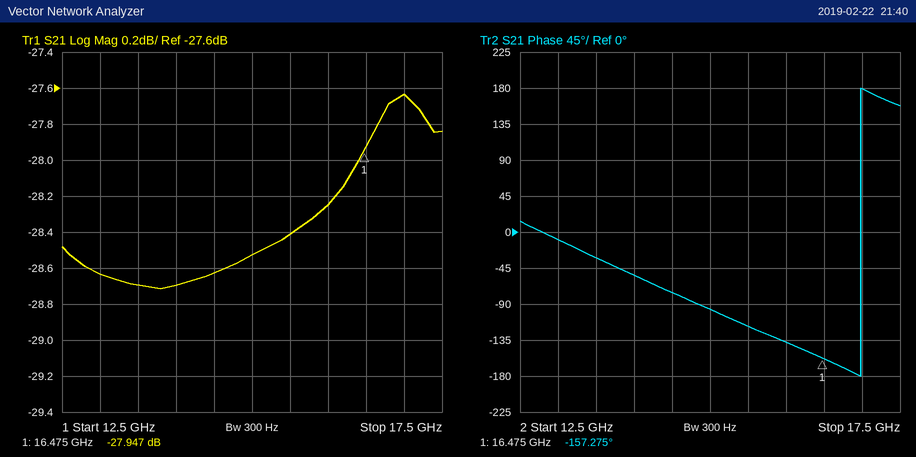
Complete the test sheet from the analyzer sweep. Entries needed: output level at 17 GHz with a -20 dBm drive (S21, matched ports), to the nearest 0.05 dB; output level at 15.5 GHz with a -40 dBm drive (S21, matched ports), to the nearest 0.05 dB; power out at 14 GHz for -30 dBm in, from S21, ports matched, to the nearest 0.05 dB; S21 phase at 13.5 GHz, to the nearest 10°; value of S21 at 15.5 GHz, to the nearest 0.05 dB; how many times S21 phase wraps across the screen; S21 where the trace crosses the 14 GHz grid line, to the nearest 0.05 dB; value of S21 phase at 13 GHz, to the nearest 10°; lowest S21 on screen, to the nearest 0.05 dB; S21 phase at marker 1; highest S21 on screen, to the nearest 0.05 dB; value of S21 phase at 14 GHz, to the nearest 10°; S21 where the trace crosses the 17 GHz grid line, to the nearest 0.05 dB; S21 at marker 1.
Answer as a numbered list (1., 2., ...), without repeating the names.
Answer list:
1. -47.65 dBm
2. -68.40 dBm
3. -58.70 dBm
4. -30°
5. -28.40 dB
6. 1
7. -28.70 dB
8. -10°
9. -28.70 dB
10. -157.275°
11. -27.65 dB
12. -50°
13. -27.65 dB
14. -27.947 dB
